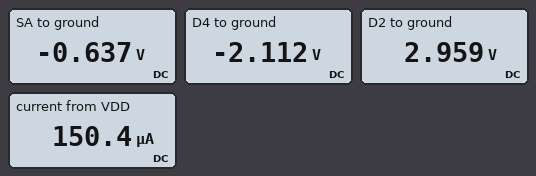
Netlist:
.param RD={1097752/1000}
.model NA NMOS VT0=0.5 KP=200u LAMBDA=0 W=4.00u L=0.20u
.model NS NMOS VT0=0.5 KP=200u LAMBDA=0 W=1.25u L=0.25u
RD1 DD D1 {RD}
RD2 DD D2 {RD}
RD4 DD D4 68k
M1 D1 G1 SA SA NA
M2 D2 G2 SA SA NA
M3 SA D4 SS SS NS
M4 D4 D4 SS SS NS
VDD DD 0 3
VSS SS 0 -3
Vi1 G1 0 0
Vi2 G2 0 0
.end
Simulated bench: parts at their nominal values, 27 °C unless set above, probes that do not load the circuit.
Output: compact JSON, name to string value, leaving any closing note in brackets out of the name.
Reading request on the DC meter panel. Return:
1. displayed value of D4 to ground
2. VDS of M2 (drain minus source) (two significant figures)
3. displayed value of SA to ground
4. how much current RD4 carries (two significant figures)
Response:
{"displayed value of D4 to ground": "-2.112 V", "VDS of M2 (drain minus source)": "3.6 V", "displayed value of SA to ground": "-0.637 V", "how much current RD4 carries": "75 µA"}
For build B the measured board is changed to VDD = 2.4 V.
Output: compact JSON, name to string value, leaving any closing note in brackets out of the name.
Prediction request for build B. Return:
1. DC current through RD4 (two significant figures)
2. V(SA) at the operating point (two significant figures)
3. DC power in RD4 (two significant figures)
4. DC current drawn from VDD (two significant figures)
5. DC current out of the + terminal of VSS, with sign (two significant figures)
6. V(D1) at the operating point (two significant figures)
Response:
{"DC current through RD4": "67 µA", "V(SA) at the operating point": "-630 mV", "DC power in RD4": "300 µW", "DC current drawn from VDD": "130 µA", "DC current out of the + terminal of VSS, with sign": "-130 µA", "V(D1) at the operating point": "2.4 V"}
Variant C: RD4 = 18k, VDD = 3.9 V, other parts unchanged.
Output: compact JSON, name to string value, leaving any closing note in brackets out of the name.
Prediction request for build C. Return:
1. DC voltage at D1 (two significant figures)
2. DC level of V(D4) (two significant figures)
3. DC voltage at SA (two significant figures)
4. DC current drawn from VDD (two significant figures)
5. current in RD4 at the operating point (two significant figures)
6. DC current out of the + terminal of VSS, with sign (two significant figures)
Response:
{"DC voltage at D1": "3.7 V", "DC level of V(D4)": "-1.7 V", "DC voltage at SA": "-780 mV", "DC current drawn from VDD": "620 µA", "current in RD4 at the operating point": "310 µA", "DC current out of the + terminal of VSS, with sign": "-620 µA"}
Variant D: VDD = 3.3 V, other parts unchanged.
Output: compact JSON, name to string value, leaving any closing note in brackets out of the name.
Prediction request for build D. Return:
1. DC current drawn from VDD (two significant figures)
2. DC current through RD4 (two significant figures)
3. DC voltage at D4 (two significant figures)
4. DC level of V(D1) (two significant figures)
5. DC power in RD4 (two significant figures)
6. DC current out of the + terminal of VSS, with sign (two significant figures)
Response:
{"DC current drawn from VDD": "160 µA", "DC current through RD4": "79 µA", "DC voltage at D4": "-2.1 V", "DC level of V(D1)": "3.3 V", "DC power in RD4": "430 µW", "DC current out of the + terminal of VSS, with sign": "-160 µA"}
